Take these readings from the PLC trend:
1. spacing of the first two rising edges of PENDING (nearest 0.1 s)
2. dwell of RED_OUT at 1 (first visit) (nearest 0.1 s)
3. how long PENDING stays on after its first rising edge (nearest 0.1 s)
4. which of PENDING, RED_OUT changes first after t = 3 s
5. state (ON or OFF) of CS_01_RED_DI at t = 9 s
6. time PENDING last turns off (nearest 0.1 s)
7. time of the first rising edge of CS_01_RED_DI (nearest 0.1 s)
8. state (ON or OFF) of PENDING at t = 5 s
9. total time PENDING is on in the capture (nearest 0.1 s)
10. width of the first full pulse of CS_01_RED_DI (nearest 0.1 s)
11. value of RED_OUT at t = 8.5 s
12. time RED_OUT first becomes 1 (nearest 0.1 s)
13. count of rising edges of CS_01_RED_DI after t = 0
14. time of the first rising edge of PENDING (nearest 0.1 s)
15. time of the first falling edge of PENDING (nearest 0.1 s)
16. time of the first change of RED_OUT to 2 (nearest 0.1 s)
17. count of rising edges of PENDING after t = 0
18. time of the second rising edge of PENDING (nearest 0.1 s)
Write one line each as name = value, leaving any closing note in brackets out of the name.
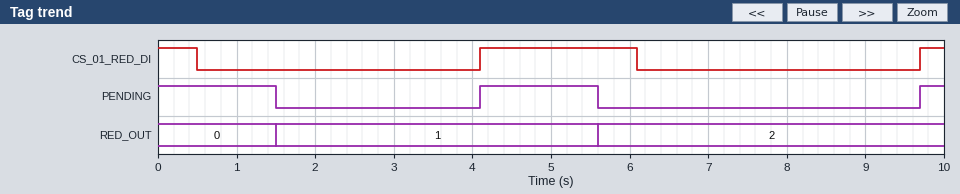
spacing of the first two rising edges of PENDING = 5.6 s
dwell of RED_OUT at 1 (first visit) = 4.1 s
how long PENDING stays on after its first rising edge = 1.5 s
which of PENDING, RED_OUT changes first after t = 3 s = PENDING
state (ON or OFF) of CS_01_RED_DI at t = 9 s = OFF
time PENDING last turns off = 5.6 s
time of the first rising edge of CS_01_RED_DI = 4.1 s
state (ON or OFF) of PENDING at t = 5 s = ON
total time PENDING is on in the capture = 3.3 s
width of the first full pulse of CS_01_RED_DI = 2.0 s
value of RED_OUT at t = 8.5 s = 2
time RED_OUT first becomes 1 = 1.5 s
count of rising edges of CS_01_RED_DI after t = 0 = 2
time of the first rising edge of PENDING = 4.1 s
time of the first falling edge of PENDING = 1.5 s
time of the first change of RED_OUT to 2 = 5.6 s
count of rising edges of PENDING after t = 0 = 2
time of the second rising edge of PENDING = 9.7 s
